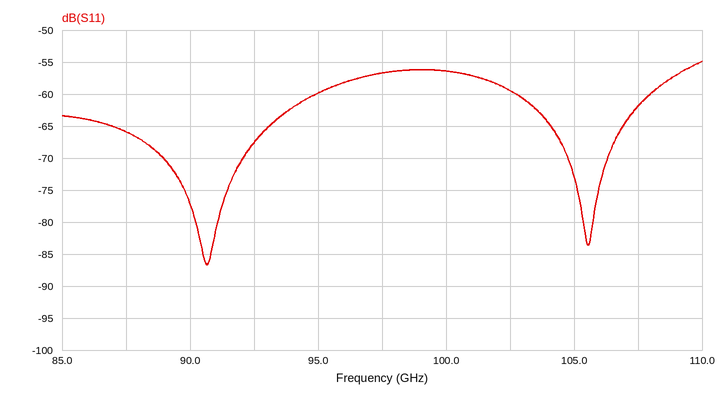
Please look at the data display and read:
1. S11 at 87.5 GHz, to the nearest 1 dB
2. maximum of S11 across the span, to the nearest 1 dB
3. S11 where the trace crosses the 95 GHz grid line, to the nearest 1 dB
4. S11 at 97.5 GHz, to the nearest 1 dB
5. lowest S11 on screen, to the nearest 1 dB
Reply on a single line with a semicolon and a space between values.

-66 dB; -55 dB; -60 dB; -57 dB; -87 dB
